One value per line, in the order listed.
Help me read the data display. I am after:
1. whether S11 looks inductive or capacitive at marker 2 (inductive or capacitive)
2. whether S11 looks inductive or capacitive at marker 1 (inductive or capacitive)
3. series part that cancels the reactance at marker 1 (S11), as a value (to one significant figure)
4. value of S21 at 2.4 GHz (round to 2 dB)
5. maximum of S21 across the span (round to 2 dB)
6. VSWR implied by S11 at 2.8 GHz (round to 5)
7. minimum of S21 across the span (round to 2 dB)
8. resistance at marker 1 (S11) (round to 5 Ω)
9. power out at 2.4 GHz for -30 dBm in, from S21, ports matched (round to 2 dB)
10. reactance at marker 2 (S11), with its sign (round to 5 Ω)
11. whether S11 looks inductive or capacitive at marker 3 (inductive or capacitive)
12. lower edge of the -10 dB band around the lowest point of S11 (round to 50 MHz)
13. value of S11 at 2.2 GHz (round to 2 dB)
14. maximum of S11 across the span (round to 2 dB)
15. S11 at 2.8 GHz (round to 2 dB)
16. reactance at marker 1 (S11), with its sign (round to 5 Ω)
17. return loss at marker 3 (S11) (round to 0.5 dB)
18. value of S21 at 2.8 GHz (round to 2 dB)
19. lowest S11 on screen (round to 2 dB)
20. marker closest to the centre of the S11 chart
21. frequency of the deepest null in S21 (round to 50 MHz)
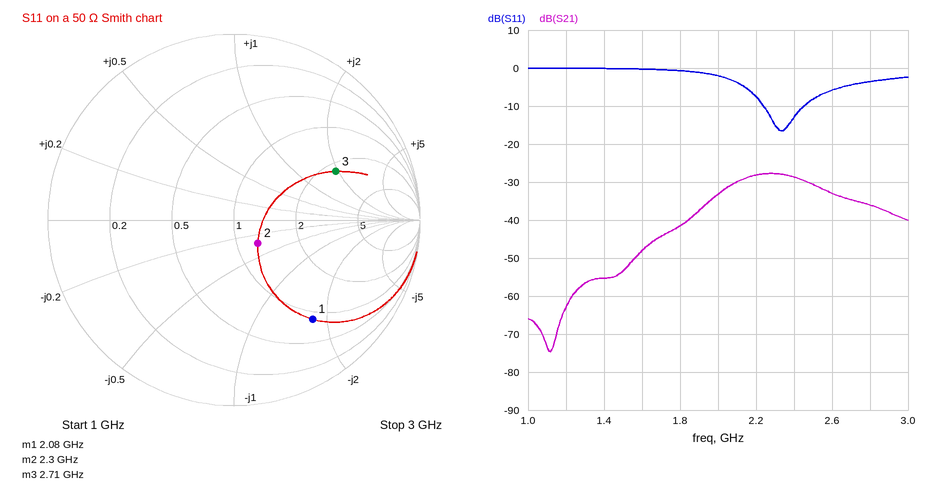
capacitive
capacitive
7 nH
-28 dB
-28 dB
5
-74 dB
45 Ω
-58 dBm
-15 Ω
inductive
2.25 GHz
-8 dB
0 dB
-4 dB
-85 Ω
4.5 dB
-36 dB
-16 dB
marker 2
1.10 GHz
